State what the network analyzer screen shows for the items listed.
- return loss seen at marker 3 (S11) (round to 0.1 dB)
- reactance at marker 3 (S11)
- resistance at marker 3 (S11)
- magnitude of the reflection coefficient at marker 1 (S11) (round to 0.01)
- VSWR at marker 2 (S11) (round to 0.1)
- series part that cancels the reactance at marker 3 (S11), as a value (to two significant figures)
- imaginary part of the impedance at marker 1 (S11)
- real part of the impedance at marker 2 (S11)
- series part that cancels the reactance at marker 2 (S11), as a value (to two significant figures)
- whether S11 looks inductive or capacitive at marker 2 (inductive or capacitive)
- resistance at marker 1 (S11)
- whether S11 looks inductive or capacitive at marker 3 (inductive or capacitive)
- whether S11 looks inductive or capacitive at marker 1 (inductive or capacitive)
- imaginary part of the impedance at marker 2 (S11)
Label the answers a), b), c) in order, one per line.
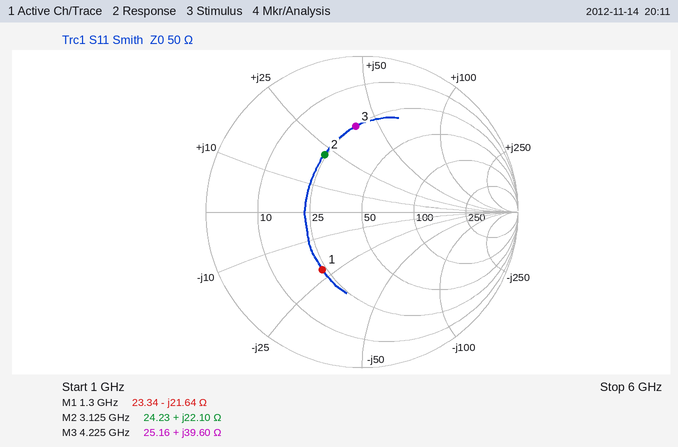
a) 5.2 dB
b) +39.60 Ω
c) 25.16 Ω
d) 0.45
e) 2.6
f) 950 fF
g) -21.64 Ω
h) 24.23 Ω
i) 2.3 pF
j) inductive
k) 23.34 Ω
l) inductive
m) capacitive
n) +22.10 Ω
